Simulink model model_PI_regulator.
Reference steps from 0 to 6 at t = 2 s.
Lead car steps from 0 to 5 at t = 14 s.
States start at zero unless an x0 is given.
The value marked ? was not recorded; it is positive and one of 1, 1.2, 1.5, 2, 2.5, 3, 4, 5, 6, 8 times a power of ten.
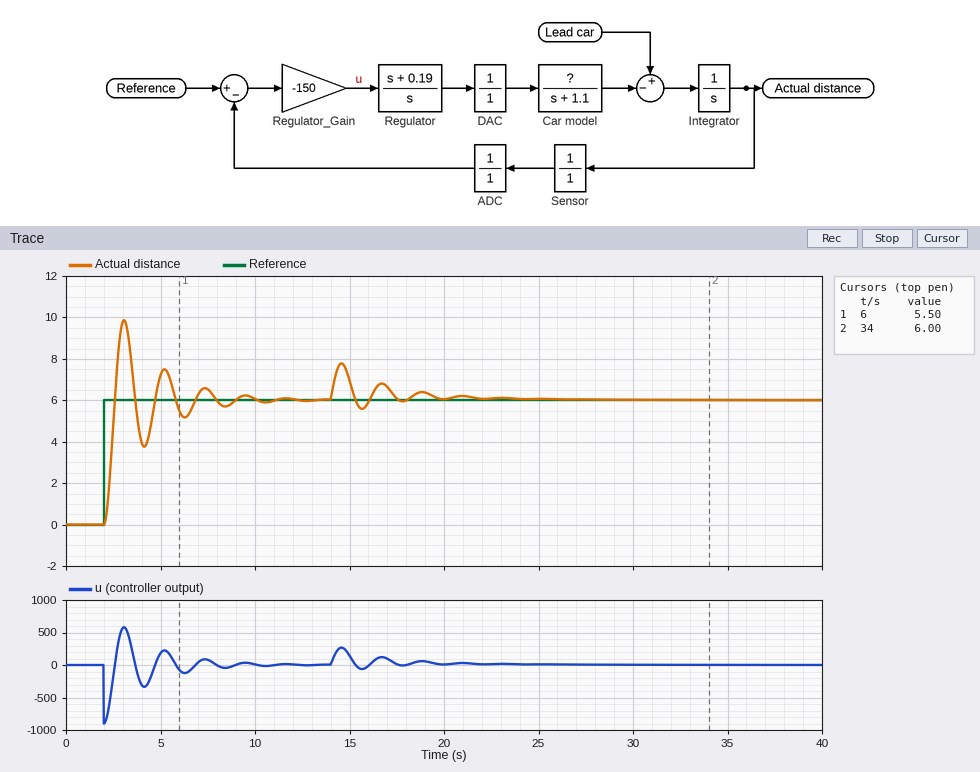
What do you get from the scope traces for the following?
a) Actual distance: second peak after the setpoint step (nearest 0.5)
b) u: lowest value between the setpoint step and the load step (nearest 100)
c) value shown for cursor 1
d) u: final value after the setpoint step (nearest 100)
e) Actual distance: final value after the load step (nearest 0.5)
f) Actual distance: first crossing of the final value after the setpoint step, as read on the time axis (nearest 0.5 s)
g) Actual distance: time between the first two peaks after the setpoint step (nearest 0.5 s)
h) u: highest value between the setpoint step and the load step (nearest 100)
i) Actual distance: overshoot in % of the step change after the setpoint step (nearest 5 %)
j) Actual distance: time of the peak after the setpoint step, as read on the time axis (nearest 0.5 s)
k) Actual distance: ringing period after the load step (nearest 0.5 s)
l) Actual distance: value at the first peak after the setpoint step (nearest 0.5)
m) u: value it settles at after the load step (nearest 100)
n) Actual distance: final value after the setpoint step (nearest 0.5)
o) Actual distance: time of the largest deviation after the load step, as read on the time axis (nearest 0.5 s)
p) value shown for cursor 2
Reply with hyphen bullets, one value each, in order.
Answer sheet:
- 7.5
- -900
- 5.50
- 0
- 6.0
- 2.5 s
- 2.0 s
- 600
- 65 %
- 3.0 s
- 2.0 s
- 10.0
- 0
- 6.0
- 14.5 s
- 6.00
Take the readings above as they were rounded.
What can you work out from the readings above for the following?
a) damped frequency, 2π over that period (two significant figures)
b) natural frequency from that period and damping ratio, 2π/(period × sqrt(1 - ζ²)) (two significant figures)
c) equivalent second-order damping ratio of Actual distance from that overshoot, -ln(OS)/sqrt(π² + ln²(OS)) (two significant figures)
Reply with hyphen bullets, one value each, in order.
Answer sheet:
- 3.1 rad/s
- 3.2 rad/s
- 0.14
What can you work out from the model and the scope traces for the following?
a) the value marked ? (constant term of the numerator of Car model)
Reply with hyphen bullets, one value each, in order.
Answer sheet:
- 0.06
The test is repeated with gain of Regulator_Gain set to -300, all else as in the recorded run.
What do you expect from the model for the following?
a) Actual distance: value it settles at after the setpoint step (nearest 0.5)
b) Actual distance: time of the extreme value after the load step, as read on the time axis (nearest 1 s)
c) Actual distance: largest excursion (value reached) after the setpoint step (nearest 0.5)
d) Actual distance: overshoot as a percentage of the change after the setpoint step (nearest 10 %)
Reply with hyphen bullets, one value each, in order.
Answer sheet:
- 6.0
- 14 s
- 10.5
- 70 %
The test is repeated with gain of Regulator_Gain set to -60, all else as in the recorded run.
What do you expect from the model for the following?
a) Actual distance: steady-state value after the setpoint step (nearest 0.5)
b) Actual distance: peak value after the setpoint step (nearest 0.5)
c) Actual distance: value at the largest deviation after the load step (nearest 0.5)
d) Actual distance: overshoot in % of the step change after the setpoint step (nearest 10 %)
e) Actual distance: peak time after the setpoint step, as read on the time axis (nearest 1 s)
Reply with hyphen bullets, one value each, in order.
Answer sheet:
- 6.0
- 9.0
- 9.0
- 50 %
- 4 s
